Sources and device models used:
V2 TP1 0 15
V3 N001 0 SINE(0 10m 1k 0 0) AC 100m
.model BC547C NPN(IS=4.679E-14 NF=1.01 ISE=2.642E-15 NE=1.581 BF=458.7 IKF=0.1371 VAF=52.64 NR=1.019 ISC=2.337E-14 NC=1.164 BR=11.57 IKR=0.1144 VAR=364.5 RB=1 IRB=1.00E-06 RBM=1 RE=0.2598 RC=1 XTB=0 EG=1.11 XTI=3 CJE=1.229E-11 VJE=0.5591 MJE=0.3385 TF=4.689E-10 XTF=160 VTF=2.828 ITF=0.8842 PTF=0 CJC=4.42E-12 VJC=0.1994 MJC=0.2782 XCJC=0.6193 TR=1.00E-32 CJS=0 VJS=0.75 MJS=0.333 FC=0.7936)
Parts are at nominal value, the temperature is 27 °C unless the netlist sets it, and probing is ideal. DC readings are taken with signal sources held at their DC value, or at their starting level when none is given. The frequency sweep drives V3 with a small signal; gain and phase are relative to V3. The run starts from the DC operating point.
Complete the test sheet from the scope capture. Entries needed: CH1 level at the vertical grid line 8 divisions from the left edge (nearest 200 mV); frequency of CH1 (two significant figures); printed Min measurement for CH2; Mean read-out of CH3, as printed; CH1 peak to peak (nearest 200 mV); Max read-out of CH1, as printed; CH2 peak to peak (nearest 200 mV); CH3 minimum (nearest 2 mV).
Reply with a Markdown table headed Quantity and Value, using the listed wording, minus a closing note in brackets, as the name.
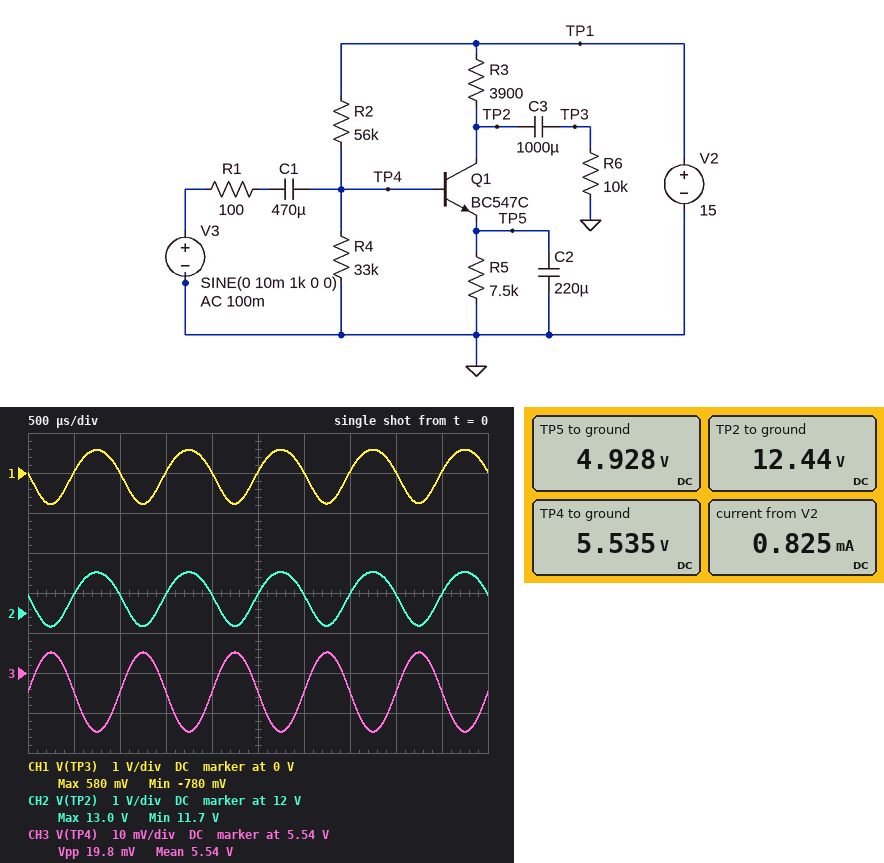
| Quantity | Value |
|---|---|
| CH1 level at the vertical grid line 8 divisions from the left edge | 0 V |
| frequency of CH1 | 1.0 kHz |
| printed Min measurement for CH2 | 11.7 V |
| Mean read-out of CH3, as printed | 5.54 V |
| CH1 peak to peak | 1.4 V |
| Max read-out of CH1, as printed | 580 mV |
| CH2 peak to peak | 1.4 V |
| CH3 minimum | 5.526 V |
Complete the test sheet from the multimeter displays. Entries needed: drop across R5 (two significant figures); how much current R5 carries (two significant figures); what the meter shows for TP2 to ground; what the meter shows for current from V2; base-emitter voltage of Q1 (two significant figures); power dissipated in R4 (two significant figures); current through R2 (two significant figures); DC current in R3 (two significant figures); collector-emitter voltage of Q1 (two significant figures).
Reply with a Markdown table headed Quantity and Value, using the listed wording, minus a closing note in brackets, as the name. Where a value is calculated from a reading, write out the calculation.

| Quantity | Value |
|---|---|
| drop across R5 | 4.928 V = 4.9 V |
| how much current R5 carries | (4.928 V) / 7.5 kΩ = 660 µA |
| what the meter shows for TP2 to ground | 12.44 V |
| what the meter shows for current from V2 | 0.825 mA |
| base-emitter voltage of Q1 | 5.535 V - 4.928 V = 610 mV |
| power dissipated in R4 | (5.535 V)^2 / 33 kΩ = 930 µW |
| current through R2 | (15 V - 5.535 V) / 56 kΩ = 170 µA |
| DC current in R3 | (15 V - 12.44 V) / 3.9 kΩ = 660 µA |
| collector-emitter voltage of Q1 | 12.44 V - 4.928 V = 7.5 V |
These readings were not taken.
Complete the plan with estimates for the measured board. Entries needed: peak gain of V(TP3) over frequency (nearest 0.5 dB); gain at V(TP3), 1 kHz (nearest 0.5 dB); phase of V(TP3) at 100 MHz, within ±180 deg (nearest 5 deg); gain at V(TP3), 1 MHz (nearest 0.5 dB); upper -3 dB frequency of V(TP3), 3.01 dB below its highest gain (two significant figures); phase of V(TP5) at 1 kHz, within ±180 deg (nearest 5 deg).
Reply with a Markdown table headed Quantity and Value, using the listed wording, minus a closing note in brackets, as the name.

| Quantity | Value |
|---|---|
| peak gain of V(TP3) over frequency | 36.5 dB |
| gain at V(TP3), 1 kHz | 36.5 dB |
| phase of V(TP3) at 100 MHz, within ±180 deg | 60 deg |
| gain at V(TP3), 1 MHz | 36.5 dB |
| upper -3 dB frequency of V(TP3), 3.01 dB below its highest gain | 8.4 MHz |
| phase of V(TP5) at 1 kHz, within ±180 deg | -90 deg |
